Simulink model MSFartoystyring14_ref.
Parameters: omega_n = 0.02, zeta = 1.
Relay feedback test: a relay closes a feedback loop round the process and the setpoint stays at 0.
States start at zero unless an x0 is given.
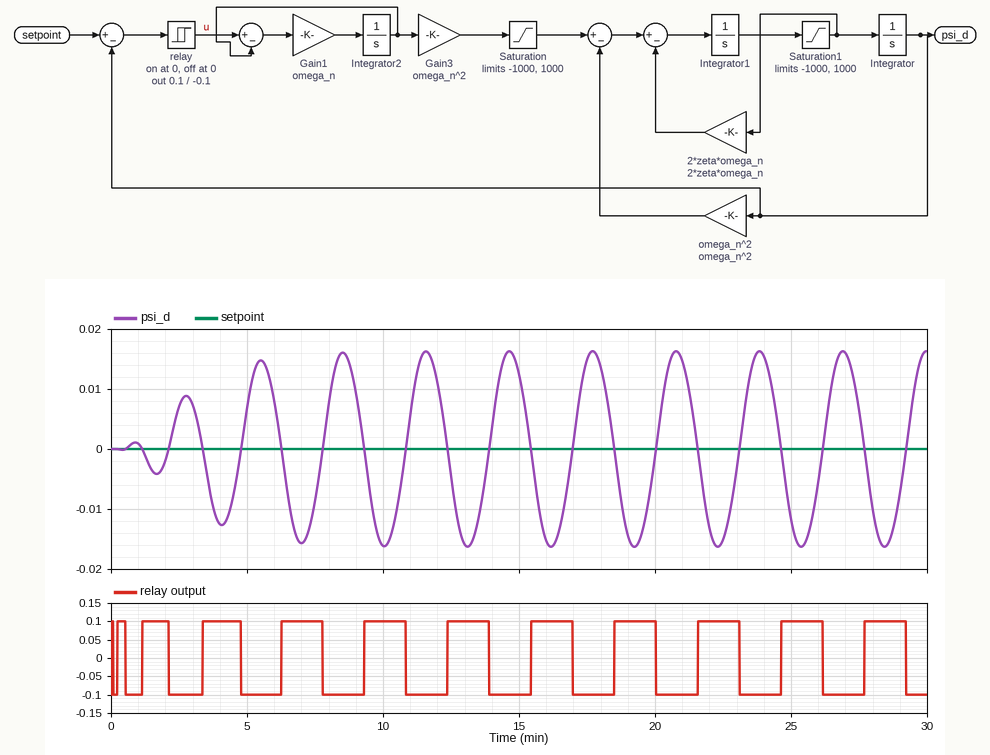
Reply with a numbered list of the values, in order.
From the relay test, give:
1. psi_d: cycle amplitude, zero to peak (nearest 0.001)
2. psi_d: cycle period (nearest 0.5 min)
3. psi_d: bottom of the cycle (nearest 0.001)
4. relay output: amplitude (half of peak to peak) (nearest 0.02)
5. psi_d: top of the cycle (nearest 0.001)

1. 0.016
2. 3.0 min
3. -0.016
4. 0.10
5. 0.016
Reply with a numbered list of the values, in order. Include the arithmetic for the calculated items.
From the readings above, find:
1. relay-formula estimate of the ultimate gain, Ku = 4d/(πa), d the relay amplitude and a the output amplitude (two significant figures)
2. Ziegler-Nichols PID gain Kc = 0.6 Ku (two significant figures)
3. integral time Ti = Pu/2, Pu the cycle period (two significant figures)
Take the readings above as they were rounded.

1. 4 × 0.1 / (π × 0.016) = 8.0
2. 0.6 × 8 = 4.8
3. 3 / 2 = 1.5 min
